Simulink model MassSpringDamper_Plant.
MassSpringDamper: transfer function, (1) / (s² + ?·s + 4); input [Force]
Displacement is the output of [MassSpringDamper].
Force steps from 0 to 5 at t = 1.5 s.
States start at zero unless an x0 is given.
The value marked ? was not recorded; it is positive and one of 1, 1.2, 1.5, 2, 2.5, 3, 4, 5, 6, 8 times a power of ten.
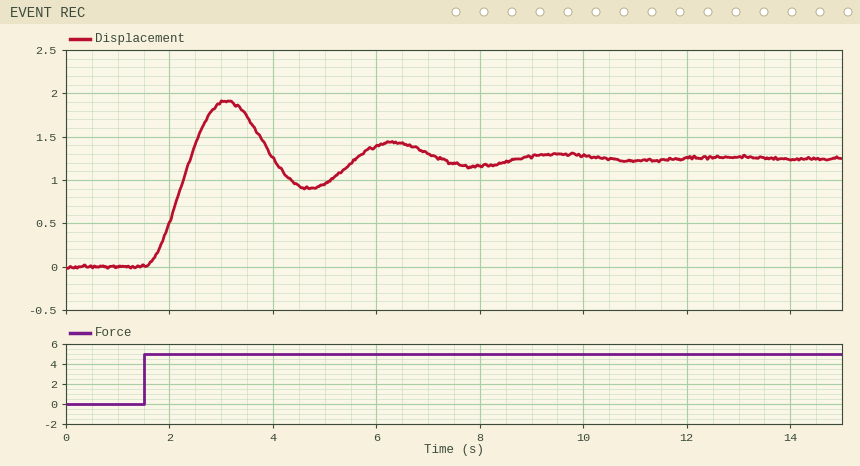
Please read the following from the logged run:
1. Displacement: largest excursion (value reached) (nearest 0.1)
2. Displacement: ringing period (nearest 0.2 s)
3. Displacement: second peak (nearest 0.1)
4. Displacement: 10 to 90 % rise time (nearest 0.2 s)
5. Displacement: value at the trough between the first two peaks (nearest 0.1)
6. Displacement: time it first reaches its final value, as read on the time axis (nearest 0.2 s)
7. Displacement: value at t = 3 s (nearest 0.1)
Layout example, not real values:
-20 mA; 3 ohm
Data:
1.9; 3.2 s; 1.4; 0.6 s; 0.9; 2.4 s; 1.9
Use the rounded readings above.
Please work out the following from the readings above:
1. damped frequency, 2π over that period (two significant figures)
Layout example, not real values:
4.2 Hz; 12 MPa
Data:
2.0 rad/s
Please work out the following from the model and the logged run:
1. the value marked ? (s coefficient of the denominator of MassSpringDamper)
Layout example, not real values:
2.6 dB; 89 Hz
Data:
0.8
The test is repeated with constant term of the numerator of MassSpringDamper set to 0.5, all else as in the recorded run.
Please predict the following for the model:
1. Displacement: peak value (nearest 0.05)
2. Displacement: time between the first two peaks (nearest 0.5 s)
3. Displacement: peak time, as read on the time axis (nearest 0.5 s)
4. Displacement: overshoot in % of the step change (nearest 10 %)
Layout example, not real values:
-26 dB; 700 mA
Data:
0.95; 3.0 s; 3.0 s; 50 %
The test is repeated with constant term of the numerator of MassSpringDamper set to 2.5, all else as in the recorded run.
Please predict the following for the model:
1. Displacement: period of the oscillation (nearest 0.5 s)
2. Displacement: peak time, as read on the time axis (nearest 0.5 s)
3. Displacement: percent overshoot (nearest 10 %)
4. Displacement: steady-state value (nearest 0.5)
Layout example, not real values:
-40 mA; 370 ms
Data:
3.0 s; 3.0 s; 50 %; 3.0
